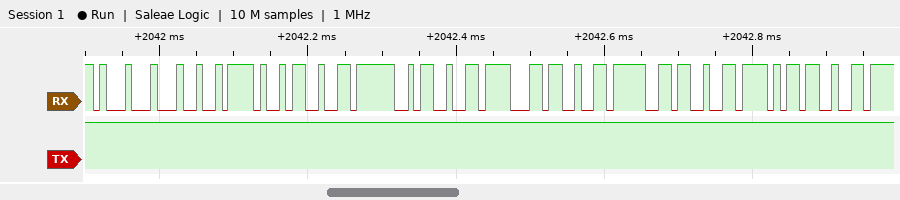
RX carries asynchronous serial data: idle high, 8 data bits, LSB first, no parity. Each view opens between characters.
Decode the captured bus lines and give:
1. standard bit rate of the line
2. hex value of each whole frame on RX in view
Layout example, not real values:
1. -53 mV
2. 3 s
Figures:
1. 115200 baud
2. 11, 24, 2F, 93, 3F, 93, 8F, 93, 9F, 93, AF, 93
